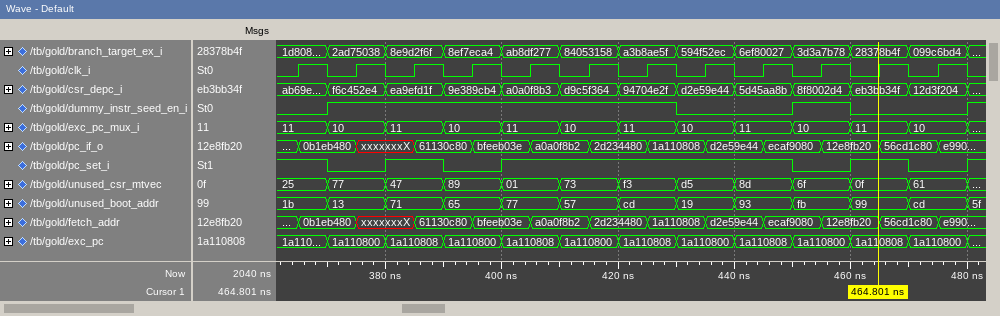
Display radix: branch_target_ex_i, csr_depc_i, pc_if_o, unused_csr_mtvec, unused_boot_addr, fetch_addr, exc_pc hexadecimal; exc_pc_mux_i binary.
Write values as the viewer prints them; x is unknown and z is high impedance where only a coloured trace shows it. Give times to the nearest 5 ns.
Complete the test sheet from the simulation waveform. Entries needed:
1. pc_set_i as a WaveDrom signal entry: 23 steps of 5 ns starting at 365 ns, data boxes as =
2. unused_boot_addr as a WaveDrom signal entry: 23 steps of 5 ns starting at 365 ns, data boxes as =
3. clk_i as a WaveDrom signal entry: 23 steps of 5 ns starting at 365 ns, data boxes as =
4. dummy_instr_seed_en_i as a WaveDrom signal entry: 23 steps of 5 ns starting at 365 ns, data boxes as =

{name: 'pc_set_i', wave: '10.1.0.1.........0.1.0.'}
{name: 'unused_boot_addr', wave: '==.=.=.=.=.=.=.=.=.=.=.', data: '1b 13 71 65 77 57 cd 19 93 fb 99 cd'}
{name: 'clk_i', wave: '10101010101010101010101'}
{name: 'dummy_instr_seed_en_i', wave: '01...........0...1.0...'}
